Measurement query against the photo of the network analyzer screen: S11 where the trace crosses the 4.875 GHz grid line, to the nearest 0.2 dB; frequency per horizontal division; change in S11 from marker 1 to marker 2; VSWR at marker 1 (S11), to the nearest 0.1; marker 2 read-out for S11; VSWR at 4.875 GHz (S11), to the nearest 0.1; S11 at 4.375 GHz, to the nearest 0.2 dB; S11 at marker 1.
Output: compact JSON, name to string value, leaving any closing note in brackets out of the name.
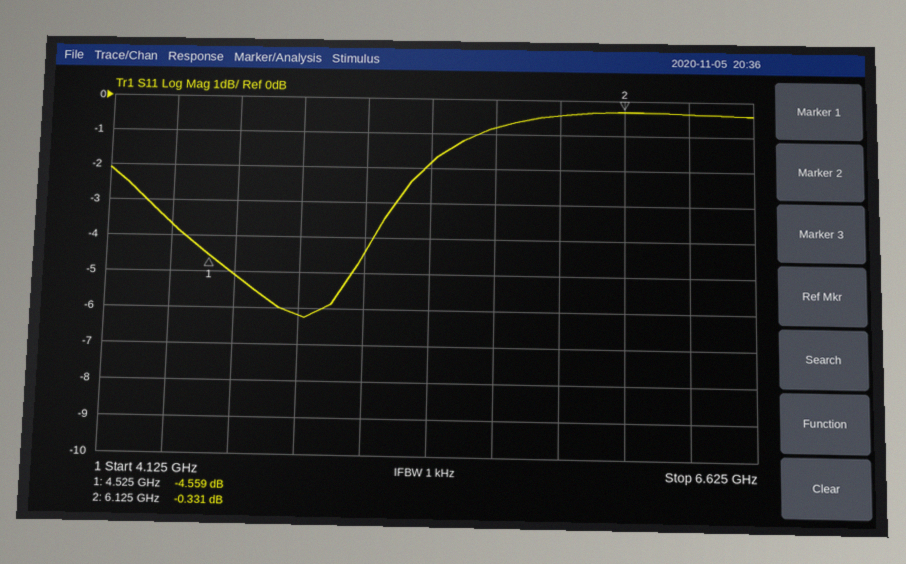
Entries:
{"S11 where the trace crosses the 4.875 GHz grid line, to the nearest 0.2 dB": "-6.2 dB", "frequency per horizontal division": "250 MHz", "change in S11 from marker 1 to marker 2": "4.228 dB", "VSWR at marker 1 (S11), to the nearest 0.1": "3.9", "marker 2 read-out for S11": "-0.331 dB", "VSWR at 4.875 GHz (S11), to the nearest 0.1": "2.9", "S11 at 4.375 GHz, to the nearest 0.2 dB": "-3.6 dB", "S11 at marker 1": "-4.559 dB"}
